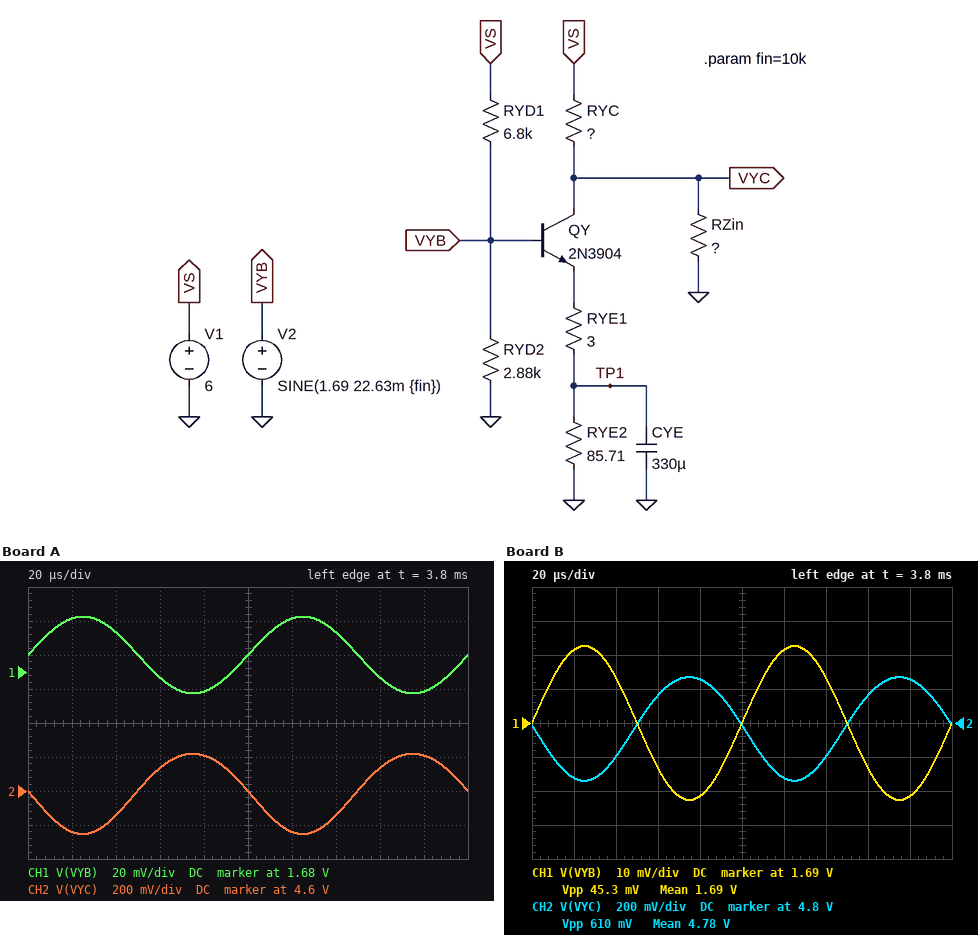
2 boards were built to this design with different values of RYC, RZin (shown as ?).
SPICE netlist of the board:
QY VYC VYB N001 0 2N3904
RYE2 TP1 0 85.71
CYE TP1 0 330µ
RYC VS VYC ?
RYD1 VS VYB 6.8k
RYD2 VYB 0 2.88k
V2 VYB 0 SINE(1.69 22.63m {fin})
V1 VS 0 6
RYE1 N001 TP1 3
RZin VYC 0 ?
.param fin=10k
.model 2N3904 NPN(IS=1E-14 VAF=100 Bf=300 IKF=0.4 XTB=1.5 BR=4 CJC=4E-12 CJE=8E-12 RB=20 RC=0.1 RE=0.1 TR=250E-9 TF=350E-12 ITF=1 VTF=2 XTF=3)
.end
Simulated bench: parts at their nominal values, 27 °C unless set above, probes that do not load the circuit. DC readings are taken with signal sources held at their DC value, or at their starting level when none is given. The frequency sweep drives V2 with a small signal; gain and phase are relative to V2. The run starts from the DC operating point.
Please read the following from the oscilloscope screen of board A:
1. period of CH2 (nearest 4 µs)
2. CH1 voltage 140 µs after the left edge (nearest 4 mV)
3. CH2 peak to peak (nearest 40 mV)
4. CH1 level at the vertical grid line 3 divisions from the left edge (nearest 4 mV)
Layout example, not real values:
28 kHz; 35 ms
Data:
100 µs; 1.704 V; 480 mV; 1.676 V
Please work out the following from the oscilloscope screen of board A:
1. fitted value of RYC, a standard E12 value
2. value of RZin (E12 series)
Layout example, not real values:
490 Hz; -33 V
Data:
68 Ω; 470 Ω
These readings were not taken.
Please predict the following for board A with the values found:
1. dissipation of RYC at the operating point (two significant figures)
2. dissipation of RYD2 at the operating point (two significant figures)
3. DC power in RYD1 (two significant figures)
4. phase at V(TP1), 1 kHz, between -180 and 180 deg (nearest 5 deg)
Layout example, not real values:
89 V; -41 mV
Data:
29 mW; 990 µW; 2.7 mW; -85 deg
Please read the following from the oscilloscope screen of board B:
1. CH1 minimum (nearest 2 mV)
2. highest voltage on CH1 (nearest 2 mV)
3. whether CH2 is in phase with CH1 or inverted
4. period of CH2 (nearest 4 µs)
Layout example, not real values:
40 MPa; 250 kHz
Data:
1.668 V; 1.712 V; inverted; 100 µs
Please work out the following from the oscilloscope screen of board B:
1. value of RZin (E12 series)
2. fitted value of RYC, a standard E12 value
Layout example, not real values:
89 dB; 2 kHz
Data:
1.2 kΩ; 82 Ω
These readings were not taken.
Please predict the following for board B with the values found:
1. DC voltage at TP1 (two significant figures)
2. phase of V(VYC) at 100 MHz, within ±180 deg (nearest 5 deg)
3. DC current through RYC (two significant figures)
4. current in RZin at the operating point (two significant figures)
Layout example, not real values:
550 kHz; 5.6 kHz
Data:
940 mV; 120 deg; 15 mA; 4.0 mA
